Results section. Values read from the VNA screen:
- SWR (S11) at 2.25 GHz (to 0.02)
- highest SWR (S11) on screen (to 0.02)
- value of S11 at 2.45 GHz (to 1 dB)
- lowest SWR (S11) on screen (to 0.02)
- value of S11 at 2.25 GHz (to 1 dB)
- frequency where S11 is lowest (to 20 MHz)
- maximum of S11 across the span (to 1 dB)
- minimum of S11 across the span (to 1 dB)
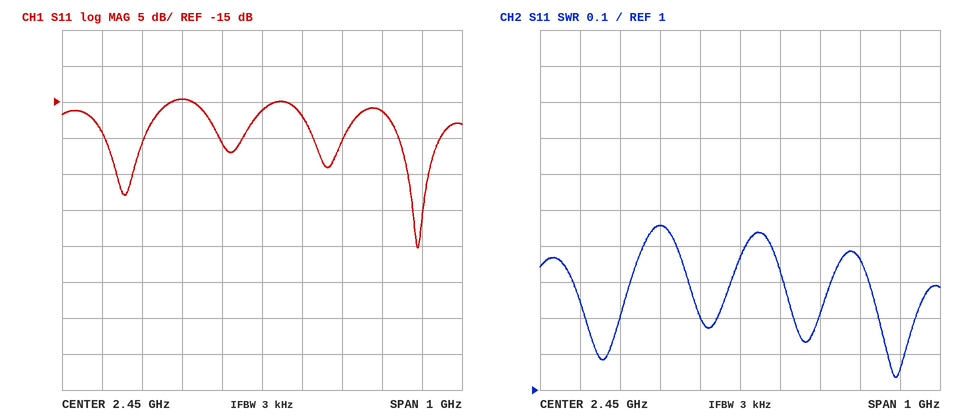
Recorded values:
1.46
1.46
-16 dB
1.04
-15 dB
2.84 GHz
-15 dB
-35 dB
